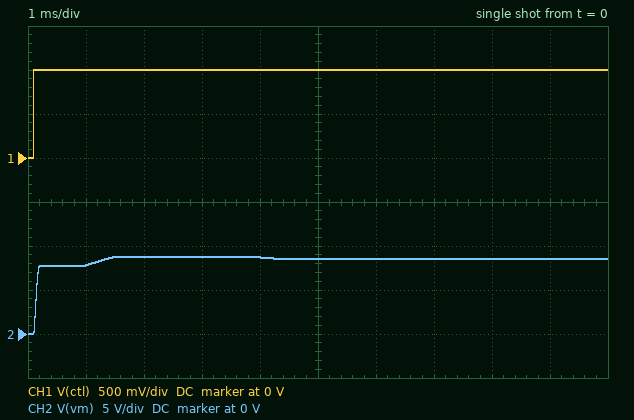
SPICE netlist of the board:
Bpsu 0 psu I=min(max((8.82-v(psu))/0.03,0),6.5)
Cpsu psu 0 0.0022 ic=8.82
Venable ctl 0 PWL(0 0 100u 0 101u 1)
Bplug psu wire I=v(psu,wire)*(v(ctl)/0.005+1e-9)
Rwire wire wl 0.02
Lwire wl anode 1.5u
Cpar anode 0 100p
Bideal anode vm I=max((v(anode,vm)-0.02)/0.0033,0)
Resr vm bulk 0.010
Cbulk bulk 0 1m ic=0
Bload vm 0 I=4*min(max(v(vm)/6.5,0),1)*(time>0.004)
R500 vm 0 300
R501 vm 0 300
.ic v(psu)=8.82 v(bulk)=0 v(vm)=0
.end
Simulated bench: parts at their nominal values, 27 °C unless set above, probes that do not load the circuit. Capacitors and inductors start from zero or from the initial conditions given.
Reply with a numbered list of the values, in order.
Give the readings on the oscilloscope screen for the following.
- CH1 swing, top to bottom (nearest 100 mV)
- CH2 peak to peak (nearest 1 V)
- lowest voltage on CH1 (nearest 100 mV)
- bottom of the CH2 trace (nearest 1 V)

1. 1.0 V
2. 9 V
3. 0 V
4. 0 V
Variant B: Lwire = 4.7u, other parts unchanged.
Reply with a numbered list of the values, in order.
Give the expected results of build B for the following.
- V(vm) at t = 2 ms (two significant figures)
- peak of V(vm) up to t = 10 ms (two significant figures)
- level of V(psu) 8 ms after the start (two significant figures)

1. 9.1 V
2. 9.2 V
3. 8.7 V
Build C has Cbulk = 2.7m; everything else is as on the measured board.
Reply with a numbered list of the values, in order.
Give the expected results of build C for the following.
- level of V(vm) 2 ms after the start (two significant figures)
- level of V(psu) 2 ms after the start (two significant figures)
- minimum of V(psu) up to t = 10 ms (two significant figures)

1. 6.4 V
2. 6.5 V
3. 3.6 V
